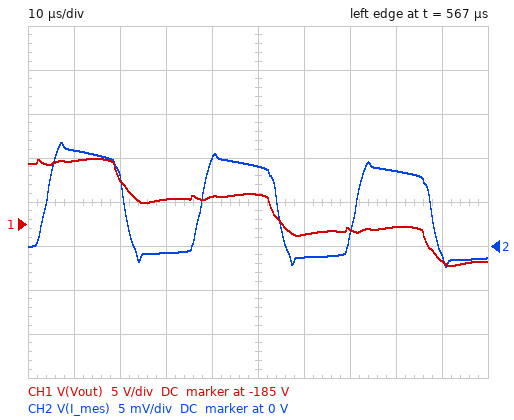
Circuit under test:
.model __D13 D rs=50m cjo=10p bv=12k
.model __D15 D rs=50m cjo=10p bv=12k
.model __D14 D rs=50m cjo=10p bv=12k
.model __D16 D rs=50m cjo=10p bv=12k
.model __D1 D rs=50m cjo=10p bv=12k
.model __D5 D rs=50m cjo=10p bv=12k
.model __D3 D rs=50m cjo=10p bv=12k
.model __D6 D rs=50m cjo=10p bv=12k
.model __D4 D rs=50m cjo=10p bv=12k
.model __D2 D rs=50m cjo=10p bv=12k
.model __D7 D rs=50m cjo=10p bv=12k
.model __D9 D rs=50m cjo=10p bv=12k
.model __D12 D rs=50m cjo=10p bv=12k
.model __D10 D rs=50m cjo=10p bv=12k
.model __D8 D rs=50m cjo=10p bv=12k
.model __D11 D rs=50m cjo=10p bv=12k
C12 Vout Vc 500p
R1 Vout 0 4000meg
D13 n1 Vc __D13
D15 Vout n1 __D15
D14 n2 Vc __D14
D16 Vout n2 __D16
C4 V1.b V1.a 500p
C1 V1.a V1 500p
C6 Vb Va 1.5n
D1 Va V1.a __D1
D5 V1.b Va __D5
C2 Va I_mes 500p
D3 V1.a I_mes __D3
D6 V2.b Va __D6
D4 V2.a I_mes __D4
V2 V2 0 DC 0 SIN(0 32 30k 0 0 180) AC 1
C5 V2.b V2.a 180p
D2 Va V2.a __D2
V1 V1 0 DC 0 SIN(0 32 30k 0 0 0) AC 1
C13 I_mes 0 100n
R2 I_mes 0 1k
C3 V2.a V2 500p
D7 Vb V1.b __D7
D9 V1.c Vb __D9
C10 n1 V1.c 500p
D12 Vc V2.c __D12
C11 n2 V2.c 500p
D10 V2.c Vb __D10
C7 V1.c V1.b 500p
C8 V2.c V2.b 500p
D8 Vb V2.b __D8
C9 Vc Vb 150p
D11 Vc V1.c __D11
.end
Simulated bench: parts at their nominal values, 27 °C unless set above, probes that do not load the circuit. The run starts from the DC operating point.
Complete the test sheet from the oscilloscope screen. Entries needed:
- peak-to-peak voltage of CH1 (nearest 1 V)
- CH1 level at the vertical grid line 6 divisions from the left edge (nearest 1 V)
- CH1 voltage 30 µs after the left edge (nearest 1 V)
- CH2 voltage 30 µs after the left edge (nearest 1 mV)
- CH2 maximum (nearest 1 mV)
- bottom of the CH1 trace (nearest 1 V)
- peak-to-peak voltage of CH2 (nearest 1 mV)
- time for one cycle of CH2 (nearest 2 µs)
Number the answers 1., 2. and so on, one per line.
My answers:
1. 12 V
2. -186 V
3. -182 V
4. -1 mV
5. 12 mV
6. -190 V
7. 14 mV
8. 34 µs
